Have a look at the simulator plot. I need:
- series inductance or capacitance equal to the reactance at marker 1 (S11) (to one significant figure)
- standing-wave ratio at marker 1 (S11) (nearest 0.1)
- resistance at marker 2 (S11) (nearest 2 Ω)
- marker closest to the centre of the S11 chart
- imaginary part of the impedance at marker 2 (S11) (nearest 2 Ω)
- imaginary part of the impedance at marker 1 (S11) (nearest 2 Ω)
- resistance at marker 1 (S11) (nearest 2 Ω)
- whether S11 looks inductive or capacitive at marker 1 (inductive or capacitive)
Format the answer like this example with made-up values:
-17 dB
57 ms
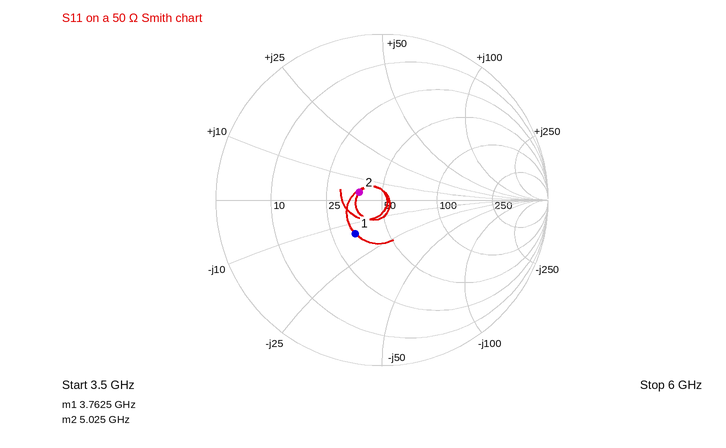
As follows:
3 pF
1.7
38 Ω
marker 2
+4 Ω
-14 Ω
34 Ω
capacitive
